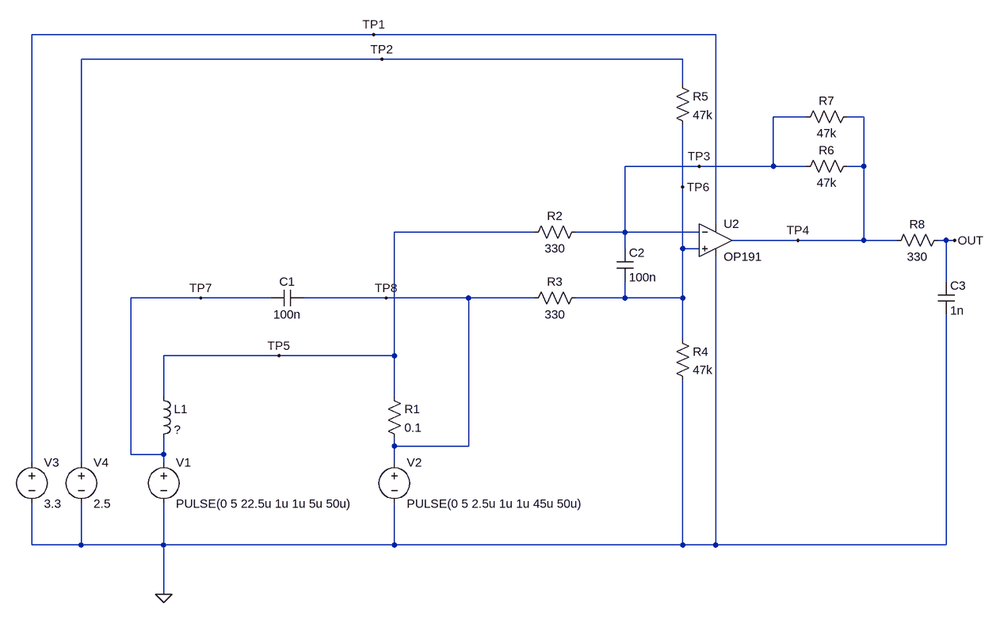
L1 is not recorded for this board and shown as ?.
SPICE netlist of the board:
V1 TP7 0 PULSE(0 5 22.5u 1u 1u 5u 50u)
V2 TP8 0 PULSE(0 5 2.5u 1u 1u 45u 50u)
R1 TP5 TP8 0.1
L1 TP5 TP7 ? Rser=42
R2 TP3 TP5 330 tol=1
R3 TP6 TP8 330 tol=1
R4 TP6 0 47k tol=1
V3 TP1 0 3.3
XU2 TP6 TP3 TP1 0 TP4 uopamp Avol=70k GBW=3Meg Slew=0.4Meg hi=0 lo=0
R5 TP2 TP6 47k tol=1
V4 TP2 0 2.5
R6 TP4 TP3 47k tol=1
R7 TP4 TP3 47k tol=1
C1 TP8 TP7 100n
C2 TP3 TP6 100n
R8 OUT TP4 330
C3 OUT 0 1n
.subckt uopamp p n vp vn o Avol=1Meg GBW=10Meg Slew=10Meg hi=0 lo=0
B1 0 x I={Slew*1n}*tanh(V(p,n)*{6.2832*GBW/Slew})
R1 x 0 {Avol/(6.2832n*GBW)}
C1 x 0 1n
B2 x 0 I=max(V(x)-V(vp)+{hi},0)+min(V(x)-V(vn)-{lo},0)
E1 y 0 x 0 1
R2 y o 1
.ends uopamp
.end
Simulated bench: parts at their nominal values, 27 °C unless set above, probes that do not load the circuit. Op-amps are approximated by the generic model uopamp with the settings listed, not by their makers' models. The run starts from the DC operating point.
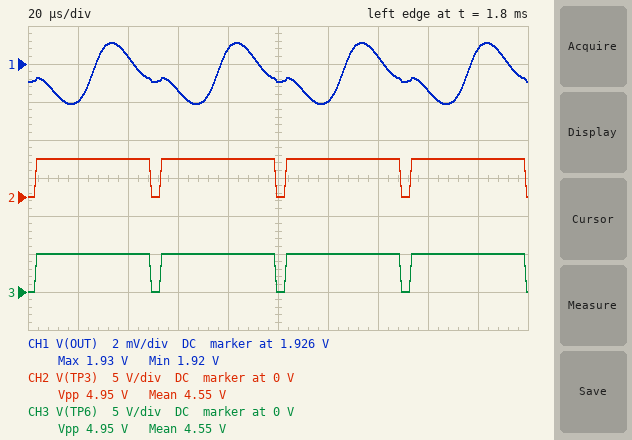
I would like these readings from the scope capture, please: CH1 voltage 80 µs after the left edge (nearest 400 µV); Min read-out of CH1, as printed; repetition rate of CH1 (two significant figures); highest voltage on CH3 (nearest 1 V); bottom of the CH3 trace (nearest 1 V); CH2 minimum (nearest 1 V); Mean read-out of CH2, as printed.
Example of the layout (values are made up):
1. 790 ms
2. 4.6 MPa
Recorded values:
1. 1.9268 V
2. 1.92 V
3. 20 kHz
4. 5 V
5. 0 V
6. 0 V
7. 4.55 V
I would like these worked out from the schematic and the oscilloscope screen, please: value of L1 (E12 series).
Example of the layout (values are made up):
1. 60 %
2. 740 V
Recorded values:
1. 5.6 mH
